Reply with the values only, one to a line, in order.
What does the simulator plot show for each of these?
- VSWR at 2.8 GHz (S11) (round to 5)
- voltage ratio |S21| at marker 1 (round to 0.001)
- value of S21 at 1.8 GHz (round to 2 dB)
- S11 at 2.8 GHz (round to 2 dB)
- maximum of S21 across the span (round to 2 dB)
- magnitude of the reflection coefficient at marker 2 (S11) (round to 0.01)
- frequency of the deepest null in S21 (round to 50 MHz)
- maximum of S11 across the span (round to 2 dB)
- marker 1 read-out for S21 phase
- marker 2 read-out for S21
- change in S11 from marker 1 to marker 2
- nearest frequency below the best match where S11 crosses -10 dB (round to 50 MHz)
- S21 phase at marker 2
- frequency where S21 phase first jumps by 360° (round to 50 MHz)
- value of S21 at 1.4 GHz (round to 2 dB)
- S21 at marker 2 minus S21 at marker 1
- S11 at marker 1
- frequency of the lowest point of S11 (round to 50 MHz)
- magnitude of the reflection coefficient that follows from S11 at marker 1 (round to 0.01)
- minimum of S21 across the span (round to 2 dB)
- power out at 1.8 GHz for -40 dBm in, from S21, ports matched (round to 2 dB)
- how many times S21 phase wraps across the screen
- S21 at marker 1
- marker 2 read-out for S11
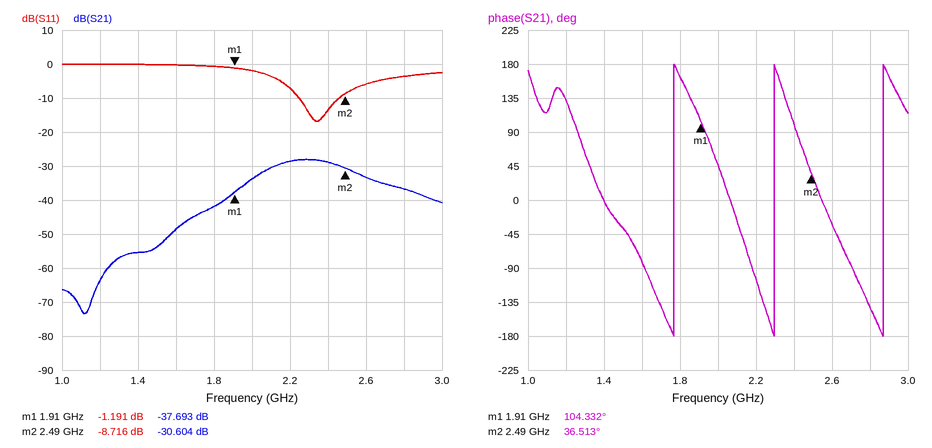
5
0.013
-42 dB
-4 dB
-28 dB
0.37
1.10 GHz
0 dB
104.332°
-30.604 dB
-7.525 dB
2.25 GHz
36.513°
1.75 GHz
-56 dB
7.089 dB
-1.191 dB
2.35 GHz
0.87
-74 dB
-82 dBm
3
-37.693 dB
-8.716 dB
